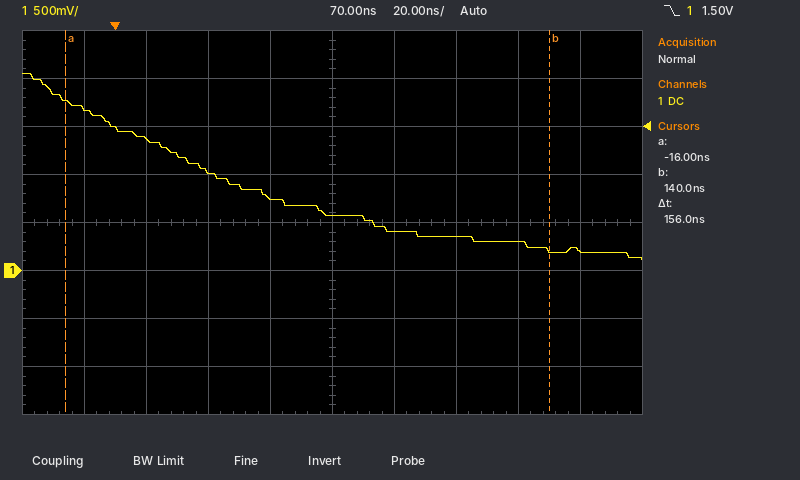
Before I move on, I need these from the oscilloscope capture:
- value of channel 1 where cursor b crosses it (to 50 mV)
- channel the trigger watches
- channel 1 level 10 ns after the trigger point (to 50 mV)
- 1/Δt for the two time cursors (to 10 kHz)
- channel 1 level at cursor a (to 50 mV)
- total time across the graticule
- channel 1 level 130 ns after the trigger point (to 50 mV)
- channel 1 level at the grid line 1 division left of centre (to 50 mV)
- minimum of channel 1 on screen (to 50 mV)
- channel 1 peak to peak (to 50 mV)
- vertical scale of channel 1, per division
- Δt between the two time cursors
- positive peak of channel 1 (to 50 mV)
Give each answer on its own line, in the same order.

200 mV
channel 1
1.35 V
6.41 MHz
1.75 V
200 ns
300 mV
750 mV
100 mV
1.95 V
500 mV
156 ns
2.05 V
